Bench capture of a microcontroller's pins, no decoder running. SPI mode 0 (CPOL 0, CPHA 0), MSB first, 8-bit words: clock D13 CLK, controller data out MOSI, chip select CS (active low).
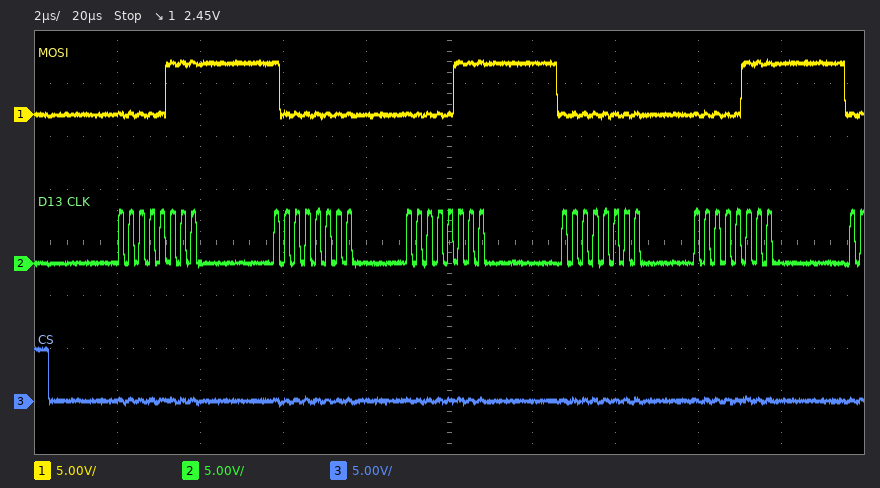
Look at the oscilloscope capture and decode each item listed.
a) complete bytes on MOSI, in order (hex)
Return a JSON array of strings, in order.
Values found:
["07 80 07 00 07"]
